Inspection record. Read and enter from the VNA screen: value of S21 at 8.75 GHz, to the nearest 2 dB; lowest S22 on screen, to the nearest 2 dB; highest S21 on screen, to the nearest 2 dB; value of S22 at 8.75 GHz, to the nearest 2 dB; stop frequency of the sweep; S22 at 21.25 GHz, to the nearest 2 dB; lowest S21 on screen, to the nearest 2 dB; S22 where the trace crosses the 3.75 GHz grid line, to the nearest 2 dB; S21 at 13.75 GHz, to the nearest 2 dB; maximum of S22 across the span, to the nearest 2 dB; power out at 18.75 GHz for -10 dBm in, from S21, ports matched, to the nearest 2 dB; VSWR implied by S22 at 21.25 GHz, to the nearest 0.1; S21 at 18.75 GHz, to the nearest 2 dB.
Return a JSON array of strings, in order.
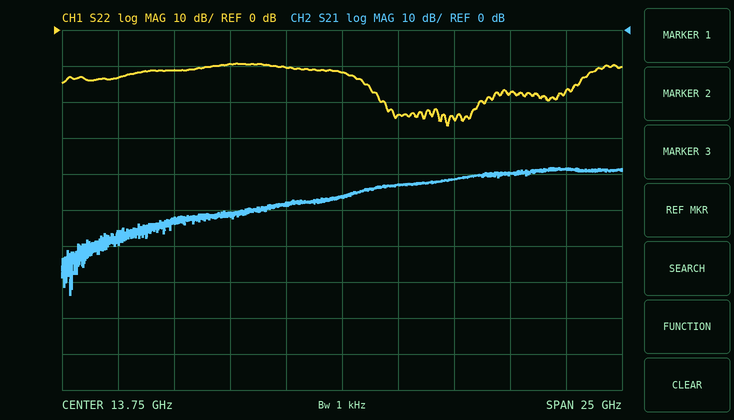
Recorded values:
["-52 dB", "-26 dB", "-38 dB", "-10 dB", "26.25 GHz", "-18 dB", "-74 dB", "-14 dB", "-46 dB", "-10 dB", "-52 dBm", "1.3", "-42 dB"]
